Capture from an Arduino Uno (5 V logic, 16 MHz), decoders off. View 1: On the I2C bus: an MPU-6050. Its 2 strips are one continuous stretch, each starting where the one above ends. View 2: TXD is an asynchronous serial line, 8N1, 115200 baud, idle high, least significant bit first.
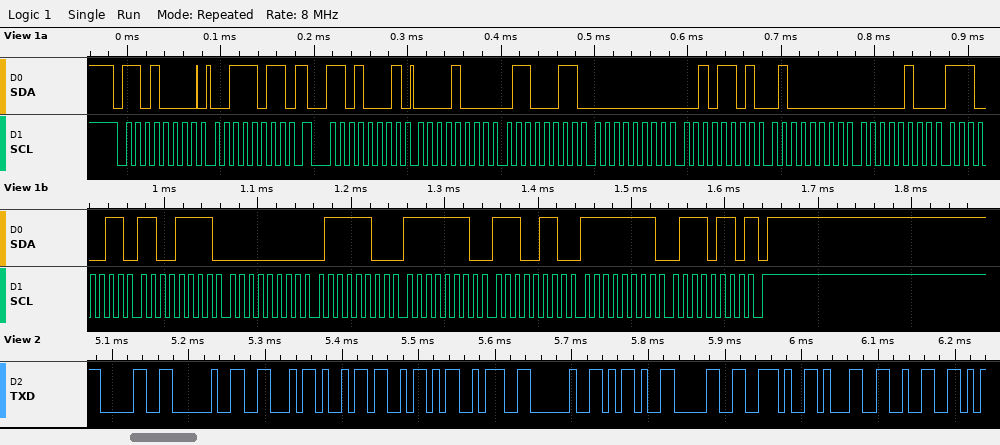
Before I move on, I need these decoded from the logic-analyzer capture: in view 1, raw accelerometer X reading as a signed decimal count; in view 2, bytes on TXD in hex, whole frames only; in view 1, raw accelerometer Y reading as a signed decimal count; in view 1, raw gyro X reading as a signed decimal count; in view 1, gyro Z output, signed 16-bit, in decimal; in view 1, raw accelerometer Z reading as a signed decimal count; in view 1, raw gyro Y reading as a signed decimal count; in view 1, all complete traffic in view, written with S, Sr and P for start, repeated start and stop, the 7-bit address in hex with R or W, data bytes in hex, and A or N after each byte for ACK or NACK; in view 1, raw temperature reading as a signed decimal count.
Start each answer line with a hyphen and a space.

- 2147
- 0x30 0x20 0x46 0x69 0x5A 0x3A 0x20 0x2D 0x30 0x2E 0x31 0x32
- 45
- 124
- -138
- 16388
- -282
- S 68W A 3B A Sr 68R A 08 A 63 A 00 A 2D A 40 A 04 A E3 A CF A 00 A 7C A FE A E6 A FF A 76 N P
- -7217
